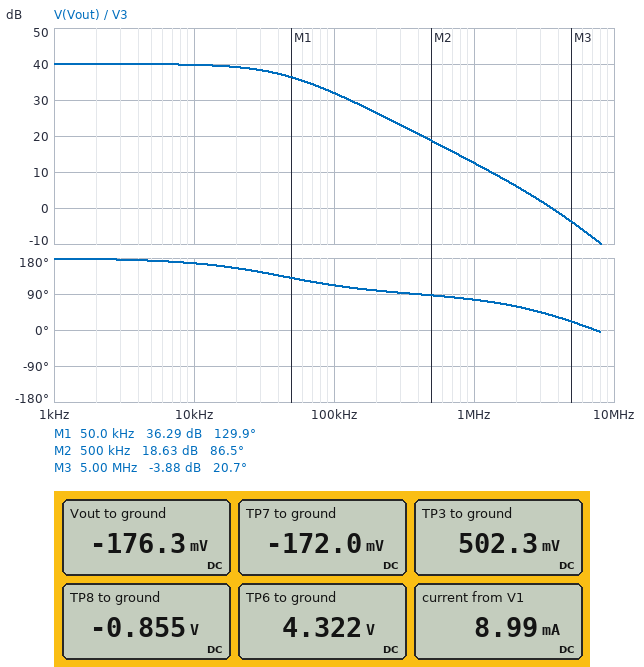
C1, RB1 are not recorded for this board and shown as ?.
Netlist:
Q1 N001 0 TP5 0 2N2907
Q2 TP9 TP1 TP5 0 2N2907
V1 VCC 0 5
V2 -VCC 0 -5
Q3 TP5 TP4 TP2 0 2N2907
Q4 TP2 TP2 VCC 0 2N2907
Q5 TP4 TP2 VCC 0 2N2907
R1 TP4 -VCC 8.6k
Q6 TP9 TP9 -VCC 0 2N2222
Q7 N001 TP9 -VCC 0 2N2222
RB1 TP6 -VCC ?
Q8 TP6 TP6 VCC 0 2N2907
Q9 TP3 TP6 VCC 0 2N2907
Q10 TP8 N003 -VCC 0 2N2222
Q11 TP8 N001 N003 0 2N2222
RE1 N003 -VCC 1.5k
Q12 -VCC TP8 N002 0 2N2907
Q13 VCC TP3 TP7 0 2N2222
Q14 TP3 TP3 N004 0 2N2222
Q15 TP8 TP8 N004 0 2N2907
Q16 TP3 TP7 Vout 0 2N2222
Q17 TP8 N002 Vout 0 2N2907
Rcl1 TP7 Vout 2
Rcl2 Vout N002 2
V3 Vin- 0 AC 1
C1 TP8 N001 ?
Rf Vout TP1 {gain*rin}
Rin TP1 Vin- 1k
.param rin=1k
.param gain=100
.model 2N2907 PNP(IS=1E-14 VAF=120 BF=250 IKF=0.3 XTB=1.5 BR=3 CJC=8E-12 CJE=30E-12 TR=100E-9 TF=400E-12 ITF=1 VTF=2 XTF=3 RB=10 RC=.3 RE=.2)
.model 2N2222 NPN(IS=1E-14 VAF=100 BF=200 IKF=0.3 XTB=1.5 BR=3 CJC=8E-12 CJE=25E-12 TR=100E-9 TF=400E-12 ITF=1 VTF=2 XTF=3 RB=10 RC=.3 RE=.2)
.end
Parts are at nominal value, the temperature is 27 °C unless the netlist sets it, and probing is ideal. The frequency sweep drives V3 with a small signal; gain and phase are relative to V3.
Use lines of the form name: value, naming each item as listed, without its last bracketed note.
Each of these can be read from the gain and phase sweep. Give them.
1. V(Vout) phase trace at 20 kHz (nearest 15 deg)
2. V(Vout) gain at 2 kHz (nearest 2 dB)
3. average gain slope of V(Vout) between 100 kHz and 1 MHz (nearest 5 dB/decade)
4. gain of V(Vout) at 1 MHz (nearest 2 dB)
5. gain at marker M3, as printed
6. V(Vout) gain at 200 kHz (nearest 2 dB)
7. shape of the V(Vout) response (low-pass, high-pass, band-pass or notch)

V(Vout) phase trace at 20 kHz: 150 deg
V(Vout) gain at 2 kHz: 40 dB
average gain slope of V(Vout) between 100 kHz and 1 MHz: -20 dB/decade
gain of V(Vout) at 1 MHz: 12 dB
gain at marker M3, as printed: -3.88 dB
V(Vout) gain at 200 kHz: 26 dB
shape of the V(Vout) response: low-pass
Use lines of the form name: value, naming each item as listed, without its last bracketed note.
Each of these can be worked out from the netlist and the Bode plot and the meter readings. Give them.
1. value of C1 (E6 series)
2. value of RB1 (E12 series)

value of C1: 680 pF
value of RB1: 3.9 kΩ
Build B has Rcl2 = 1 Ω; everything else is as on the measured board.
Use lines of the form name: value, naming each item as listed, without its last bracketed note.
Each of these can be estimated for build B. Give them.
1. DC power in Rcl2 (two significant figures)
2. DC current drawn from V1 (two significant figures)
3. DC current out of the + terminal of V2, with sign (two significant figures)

DC power in Rcl2: 5.0 µW
DC current drawn from V1: 9.1 mA
DC current out of the + terminal of V2, with sign: -9.1 mA
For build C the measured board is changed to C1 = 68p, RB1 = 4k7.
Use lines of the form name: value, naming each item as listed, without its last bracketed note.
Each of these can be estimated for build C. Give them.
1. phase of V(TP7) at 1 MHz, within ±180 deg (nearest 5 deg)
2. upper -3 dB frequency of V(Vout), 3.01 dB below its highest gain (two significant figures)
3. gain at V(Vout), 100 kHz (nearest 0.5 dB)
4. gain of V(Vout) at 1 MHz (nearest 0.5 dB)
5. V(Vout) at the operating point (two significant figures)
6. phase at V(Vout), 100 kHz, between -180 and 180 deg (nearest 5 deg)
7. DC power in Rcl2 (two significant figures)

phase of V(TP7) at 1 MHz, within ±180 deg: 100 deg
upper -3 dB frequency of V(Vout), 3.01 dB below its highest gain: 440 kHz
gain at V(Vout), 100 kHz: 40.0 dB
gain of V(Vout) at 1 MHz: 32.0 dB
V(Vout) at the operating point: -180 mV
phase at V(Vout), 100 kHz, between -180 and 180 deg: 165 deg
DC power in Rcl2: 6.7 µW
